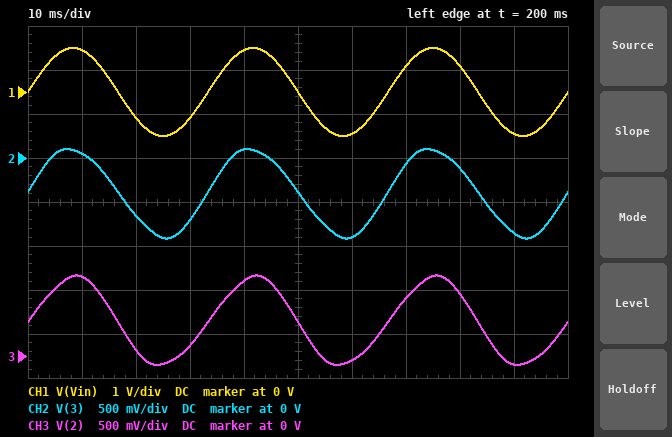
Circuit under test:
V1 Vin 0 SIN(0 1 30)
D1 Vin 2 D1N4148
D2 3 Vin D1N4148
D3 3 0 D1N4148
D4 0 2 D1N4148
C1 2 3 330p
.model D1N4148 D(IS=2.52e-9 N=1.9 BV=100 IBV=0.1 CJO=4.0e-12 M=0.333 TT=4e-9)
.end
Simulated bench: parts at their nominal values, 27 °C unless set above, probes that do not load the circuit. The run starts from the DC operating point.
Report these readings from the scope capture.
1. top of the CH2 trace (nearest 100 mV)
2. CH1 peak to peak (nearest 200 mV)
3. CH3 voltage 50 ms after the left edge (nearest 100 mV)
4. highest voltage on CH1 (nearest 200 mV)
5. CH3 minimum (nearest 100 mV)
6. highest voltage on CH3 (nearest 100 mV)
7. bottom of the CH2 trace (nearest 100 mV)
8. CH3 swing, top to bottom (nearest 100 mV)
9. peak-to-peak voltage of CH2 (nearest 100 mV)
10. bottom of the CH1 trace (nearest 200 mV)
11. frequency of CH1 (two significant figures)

100 mV
2.0 V
400 mV
1.0 V
-100 mV
900 mV
-900 mV
1.0 V
1.0 V
-1.0 V
30 Hz
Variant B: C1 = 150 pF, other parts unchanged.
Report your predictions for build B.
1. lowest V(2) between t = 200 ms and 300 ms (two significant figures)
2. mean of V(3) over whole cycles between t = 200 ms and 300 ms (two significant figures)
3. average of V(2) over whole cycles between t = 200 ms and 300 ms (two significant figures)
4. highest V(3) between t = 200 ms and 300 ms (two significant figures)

-96 mV
-380 mV
380 mV
96 mV
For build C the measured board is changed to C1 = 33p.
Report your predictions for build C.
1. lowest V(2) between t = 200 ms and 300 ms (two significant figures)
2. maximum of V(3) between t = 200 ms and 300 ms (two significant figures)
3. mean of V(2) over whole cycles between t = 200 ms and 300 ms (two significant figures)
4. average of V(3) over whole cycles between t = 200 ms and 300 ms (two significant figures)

-73 mV
73 mV
310 mV
-310 mV
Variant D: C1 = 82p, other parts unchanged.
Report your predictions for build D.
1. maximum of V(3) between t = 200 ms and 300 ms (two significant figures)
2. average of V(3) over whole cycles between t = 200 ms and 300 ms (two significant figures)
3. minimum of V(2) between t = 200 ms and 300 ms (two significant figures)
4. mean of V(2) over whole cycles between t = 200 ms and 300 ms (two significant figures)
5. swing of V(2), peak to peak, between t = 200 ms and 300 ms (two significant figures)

89 mV
-350 mV
-89 mV
350 mV
1.0 V
